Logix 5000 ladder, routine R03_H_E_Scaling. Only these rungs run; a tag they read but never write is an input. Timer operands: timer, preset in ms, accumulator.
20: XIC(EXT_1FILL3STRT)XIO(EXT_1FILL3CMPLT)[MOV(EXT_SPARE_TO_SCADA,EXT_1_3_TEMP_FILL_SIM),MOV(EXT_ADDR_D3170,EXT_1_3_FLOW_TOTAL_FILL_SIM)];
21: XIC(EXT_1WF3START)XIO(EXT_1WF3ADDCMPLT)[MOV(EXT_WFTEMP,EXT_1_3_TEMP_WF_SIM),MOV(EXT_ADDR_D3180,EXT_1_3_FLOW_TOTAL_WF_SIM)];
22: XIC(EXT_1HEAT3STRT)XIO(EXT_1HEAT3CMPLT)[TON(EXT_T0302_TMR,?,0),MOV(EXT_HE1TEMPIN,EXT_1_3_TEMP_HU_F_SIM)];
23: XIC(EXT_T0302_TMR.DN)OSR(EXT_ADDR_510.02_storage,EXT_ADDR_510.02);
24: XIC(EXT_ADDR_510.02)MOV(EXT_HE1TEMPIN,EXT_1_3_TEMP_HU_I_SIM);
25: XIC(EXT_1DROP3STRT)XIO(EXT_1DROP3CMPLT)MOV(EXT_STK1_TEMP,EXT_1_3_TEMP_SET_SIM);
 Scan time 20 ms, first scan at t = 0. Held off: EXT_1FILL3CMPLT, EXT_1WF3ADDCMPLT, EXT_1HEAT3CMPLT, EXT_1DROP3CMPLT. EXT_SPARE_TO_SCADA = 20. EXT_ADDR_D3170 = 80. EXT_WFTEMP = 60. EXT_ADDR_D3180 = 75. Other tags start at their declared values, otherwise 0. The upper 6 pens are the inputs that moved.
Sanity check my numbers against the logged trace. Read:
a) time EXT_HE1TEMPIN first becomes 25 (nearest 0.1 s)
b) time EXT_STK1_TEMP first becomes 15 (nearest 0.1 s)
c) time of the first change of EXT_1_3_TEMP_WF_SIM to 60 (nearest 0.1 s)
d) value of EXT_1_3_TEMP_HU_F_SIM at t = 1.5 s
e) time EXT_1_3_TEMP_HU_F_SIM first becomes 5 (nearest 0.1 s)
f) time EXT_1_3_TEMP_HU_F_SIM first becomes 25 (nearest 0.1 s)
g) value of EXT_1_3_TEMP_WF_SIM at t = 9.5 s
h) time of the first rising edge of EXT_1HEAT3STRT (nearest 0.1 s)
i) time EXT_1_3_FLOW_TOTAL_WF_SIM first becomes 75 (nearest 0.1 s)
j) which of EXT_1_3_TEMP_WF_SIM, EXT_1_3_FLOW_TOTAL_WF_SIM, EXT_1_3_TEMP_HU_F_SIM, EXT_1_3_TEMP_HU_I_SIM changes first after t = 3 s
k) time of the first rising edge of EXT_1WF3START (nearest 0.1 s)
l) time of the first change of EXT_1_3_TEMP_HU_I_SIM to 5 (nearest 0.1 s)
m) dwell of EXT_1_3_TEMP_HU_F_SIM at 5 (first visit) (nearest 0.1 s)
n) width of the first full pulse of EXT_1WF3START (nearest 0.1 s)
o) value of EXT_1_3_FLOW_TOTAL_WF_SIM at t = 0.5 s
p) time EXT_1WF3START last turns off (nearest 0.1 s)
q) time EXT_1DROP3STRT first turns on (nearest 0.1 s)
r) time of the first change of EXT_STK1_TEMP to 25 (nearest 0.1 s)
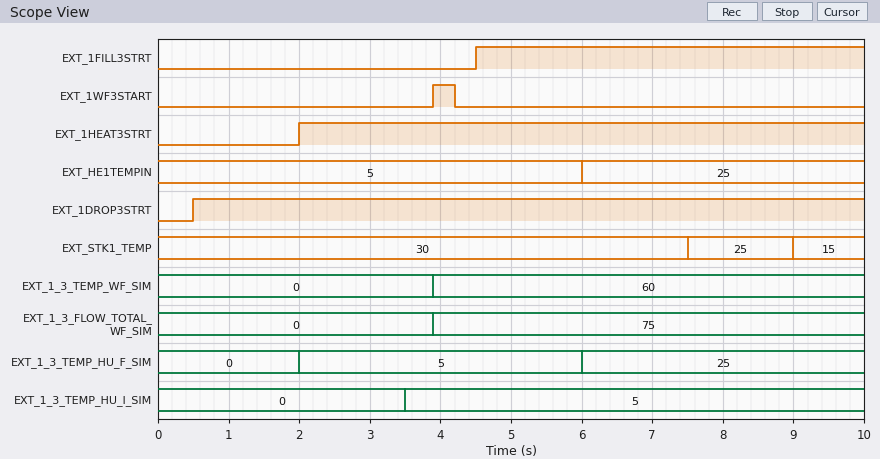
6.0 s
9.0 s
3.9 s
0
2.0 s
6.0 s
60
2.0 s
3.9 s
EXT_1_3_TEMP_HU_I_SIM
3.9 s
3.5 s
4.0 s
0.3 s
0
4.2 s
0.5 s
7.5 s
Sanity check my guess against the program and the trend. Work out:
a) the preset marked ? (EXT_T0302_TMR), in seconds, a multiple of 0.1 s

1.5 s
